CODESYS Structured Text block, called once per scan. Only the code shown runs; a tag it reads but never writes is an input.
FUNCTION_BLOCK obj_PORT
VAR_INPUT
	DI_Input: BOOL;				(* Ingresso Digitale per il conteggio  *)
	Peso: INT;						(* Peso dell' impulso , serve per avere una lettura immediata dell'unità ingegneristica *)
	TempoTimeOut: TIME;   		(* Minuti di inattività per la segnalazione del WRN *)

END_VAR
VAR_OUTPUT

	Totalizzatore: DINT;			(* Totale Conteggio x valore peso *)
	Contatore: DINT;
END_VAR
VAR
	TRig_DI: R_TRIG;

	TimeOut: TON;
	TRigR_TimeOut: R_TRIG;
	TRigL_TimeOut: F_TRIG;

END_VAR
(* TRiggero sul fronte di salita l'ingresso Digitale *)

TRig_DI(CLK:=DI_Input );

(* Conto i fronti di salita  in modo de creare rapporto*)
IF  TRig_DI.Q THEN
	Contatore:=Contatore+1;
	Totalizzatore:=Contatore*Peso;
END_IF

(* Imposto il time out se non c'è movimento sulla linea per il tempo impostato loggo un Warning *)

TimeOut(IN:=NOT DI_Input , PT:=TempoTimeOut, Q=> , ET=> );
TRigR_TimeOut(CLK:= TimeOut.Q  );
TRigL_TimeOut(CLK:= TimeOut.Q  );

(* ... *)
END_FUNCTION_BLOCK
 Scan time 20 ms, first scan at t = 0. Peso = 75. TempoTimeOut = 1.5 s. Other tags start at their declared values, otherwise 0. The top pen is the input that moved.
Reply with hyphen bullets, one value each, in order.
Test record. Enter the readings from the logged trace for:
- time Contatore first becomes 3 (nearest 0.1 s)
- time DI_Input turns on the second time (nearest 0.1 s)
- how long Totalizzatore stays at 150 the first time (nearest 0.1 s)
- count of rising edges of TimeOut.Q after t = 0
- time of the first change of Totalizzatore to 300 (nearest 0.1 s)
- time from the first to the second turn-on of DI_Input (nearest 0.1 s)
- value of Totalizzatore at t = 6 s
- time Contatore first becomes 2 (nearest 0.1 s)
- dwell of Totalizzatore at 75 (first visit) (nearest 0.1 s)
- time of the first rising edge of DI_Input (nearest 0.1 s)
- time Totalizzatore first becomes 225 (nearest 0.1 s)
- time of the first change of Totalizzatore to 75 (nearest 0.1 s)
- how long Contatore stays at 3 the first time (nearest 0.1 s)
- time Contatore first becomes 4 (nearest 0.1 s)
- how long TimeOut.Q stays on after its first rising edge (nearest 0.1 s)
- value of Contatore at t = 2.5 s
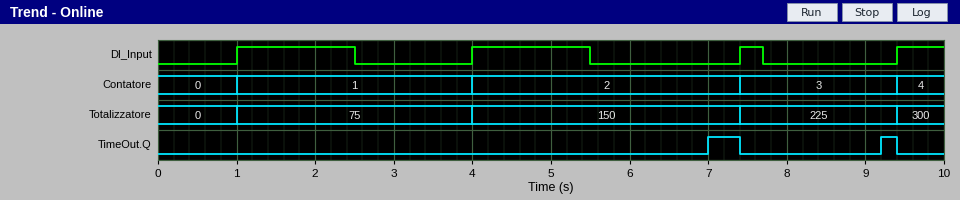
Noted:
- 7.4 s
- 4.0 s
- 3.4 s
- 2
- 9.4 s
- 3.0 s
- 150
- 4.0 s
- 3.0 s
- 1.0 s
- 7.4 s
- 1.0 s
- 2.0 s
- 9.4 s
- 0.4 s
- 1
